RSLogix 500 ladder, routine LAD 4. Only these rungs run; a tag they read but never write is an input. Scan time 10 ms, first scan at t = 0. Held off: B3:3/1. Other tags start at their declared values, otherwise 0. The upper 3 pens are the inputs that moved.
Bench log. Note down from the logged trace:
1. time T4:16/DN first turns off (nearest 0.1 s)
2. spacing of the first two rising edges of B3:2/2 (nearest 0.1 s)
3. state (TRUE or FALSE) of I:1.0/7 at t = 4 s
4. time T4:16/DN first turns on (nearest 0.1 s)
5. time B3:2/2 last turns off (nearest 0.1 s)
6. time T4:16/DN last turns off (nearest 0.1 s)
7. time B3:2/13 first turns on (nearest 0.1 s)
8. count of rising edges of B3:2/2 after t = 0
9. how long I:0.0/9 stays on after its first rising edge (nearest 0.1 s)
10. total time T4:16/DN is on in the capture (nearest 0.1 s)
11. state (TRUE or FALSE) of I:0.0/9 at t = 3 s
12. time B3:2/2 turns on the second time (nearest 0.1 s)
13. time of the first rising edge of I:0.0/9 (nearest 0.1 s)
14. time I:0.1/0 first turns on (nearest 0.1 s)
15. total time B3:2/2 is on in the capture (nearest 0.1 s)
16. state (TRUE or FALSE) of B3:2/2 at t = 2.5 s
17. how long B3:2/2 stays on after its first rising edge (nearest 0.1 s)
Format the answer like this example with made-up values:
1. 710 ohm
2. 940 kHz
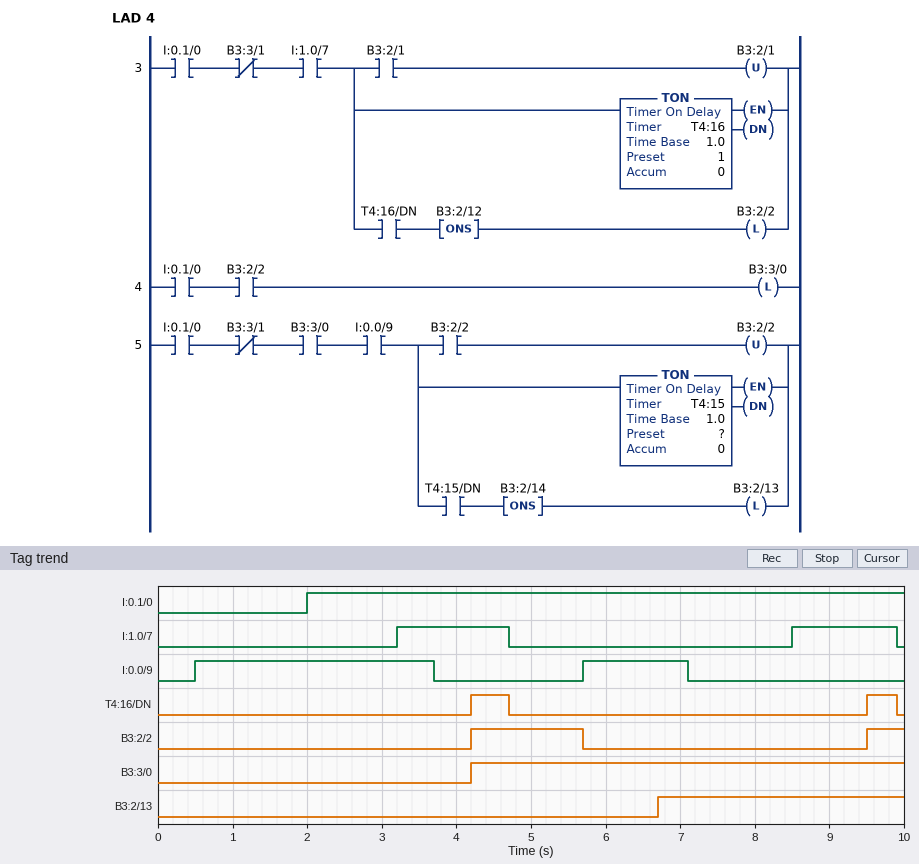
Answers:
1. 4.7 s
2. 5.3 s
3. TRUE
4. 4.2 s
5. 5.7 s
6. 9.9 s
7. 6.7 s
8. 2
9. 3.2 s
10. 0.9 s
11. TRUE
12. 9.5 s
13. 0.5 s
14. 2.0 s
15. 2.0 s
16. FALSE
17. 1.5 s
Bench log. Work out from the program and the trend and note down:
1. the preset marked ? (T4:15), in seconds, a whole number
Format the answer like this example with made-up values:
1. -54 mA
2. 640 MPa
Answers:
1. 1 s
